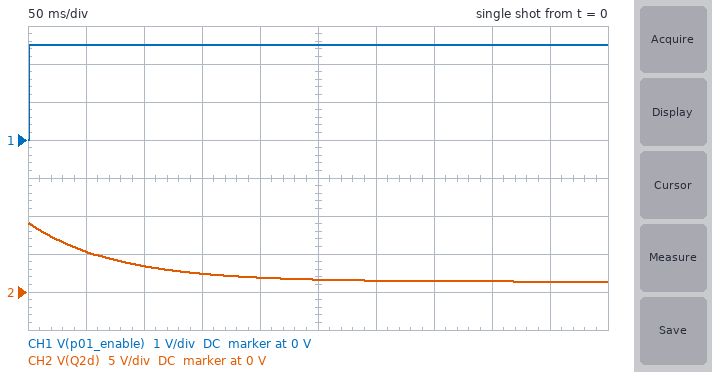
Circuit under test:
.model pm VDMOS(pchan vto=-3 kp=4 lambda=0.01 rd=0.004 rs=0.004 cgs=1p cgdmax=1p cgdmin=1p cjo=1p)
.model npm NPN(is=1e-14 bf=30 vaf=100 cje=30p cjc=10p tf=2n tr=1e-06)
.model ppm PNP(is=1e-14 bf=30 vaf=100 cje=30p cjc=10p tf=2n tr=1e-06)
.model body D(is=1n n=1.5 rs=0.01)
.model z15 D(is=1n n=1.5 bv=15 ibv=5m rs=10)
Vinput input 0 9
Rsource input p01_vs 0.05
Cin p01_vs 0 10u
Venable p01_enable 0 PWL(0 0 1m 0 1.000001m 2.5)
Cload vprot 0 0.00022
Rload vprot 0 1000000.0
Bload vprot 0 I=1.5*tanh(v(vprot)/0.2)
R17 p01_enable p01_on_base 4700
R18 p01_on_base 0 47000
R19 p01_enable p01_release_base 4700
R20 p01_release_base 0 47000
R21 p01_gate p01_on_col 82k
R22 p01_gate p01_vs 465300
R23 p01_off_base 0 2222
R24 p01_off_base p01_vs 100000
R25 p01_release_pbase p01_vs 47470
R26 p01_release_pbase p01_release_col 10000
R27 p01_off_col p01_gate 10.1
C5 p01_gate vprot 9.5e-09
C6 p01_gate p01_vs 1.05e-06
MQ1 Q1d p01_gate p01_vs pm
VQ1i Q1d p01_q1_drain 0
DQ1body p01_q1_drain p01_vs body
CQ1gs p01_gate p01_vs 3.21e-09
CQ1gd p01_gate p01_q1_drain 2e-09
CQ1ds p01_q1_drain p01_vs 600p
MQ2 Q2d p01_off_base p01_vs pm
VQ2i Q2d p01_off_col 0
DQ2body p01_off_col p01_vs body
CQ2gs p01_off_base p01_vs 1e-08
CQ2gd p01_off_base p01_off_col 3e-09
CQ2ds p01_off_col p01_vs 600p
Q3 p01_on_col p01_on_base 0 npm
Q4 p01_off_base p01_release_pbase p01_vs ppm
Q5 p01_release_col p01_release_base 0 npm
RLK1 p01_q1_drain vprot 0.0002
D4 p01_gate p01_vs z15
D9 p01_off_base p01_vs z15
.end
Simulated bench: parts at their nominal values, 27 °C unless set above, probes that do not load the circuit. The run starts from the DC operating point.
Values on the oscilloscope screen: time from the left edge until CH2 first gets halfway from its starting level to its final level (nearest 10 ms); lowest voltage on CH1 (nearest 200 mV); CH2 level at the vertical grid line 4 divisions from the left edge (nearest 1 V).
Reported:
50 ms
0 V
2 V
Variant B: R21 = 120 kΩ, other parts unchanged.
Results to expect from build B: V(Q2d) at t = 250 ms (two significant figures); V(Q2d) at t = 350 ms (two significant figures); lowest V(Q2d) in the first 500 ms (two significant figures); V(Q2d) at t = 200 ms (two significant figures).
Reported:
2.5 V
2.1 V
1.9 V
2.9 V
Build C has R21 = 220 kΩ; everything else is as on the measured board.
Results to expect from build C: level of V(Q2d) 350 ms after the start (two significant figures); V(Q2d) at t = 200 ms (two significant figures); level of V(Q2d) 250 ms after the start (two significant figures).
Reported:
3.6 V
4.7 V
4.2 V
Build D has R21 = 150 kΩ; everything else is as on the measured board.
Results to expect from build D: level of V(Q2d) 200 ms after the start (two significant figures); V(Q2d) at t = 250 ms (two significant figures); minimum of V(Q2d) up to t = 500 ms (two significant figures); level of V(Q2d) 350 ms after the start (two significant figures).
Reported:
3.5 V
3.1 V
2.3 V
2.6 V
